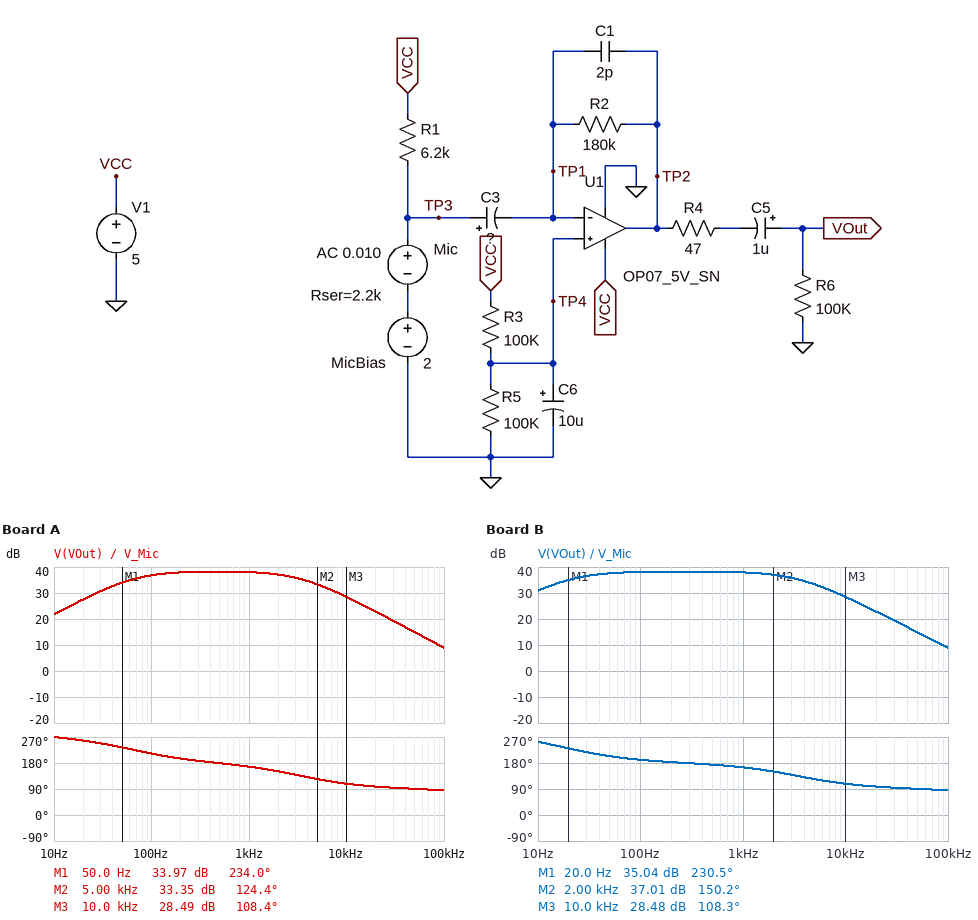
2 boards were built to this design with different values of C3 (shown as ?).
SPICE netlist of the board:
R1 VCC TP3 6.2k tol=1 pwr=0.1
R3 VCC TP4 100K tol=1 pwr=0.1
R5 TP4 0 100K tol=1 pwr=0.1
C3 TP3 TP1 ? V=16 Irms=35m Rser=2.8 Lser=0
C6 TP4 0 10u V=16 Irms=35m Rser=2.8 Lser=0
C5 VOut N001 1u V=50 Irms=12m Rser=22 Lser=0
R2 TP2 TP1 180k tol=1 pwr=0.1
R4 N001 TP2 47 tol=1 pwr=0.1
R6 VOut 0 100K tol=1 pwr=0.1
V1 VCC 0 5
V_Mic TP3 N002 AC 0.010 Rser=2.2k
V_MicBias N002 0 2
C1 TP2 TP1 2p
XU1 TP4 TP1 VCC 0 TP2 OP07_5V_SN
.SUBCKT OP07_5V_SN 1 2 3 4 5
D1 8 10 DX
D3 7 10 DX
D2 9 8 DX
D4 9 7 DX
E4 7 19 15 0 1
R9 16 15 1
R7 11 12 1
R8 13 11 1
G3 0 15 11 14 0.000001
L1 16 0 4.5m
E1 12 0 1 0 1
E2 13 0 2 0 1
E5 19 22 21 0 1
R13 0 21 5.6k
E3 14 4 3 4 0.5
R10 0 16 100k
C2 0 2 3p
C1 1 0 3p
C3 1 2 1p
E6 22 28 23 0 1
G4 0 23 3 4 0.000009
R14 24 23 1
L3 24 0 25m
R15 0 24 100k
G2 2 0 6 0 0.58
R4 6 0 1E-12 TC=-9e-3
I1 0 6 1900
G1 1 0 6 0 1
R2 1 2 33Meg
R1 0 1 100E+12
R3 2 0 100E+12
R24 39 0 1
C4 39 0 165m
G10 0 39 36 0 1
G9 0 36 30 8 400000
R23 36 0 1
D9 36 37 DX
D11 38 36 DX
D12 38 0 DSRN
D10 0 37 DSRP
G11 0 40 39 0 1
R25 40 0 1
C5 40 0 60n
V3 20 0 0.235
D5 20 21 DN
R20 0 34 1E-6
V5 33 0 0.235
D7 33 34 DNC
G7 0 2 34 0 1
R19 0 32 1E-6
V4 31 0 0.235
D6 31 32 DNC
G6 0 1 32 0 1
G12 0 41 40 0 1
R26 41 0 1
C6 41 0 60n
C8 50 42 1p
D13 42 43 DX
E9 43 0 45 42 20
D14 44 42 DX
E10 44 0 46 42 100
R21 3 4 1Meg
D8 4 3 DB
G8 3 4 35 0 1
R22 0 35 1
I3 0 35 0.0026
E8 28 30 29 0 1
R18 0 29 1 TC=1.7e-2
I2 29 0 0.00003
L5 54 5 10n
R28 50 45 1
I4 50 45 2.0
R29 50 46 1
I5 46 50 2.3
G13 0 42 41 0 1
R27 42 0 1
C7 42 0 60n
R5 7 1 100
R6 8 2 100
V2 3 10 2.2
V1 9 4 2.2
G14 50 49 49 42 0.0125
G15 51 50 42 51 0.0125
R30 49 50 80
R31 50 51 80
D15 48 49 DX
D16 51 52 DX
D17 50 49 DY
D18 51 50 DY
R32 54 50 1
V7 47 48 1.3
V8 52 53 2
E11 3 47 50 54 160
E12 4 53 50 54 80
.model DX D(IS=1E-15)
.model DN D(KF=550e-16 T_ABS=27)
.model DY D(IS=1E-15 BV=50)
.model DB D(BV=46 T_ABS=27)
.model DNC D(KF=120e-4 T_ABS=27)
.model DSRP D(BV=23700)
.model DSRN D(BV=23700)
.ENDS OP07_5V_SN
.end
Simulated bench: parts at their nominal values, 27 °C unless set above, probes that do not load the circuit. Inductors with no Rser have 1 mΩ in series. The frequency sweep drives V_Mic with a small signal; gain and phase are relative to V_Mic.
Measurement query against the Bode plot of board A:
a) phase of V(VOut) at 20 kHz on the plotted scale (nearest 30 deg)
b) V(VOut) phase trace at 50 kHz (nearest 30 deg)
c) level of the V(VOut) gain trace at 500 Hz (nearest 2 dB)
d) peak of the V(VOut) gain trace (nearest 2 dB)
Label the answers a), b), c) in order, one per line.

a) 90 deg
b) 90 deg
c) 38 dB
d) 38 dB
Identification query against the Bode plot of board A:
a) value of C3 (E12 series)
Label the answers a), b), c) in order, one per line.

a) 1.5 µF
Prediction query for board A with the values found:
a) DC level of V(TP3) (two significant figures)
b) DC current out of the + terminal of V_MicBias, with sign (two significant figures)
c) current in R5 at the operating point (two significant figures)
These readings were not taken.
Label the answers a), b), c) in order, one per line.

a) 2.8 V
b) -360 µA
c) 25 µA
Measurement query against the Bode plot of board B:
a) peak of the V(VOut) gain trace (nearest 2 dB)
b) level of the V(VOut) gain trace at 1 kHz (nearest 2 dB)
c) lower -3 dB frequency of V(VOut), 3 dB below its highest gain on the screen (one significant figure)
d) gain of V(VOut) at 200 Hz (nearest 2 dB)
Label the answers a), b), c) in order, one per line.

a) 38 dB
b) 38 dB
c) 20 Hz
d) 38 dB
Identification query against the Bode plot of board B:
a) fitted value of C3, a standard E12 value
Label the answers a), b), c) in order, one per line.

a) 4.7 µF
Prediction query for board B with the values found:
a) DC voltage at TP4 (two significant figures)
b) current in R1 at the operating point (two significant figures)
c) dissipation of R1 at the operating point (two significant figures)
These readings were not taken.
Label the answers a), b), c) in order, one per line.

a) 2.5 V
b) 360 µA
c) 790 µW
